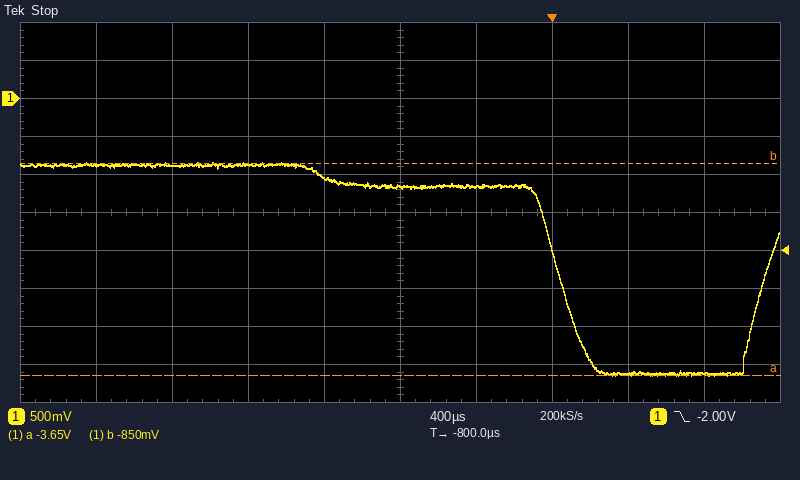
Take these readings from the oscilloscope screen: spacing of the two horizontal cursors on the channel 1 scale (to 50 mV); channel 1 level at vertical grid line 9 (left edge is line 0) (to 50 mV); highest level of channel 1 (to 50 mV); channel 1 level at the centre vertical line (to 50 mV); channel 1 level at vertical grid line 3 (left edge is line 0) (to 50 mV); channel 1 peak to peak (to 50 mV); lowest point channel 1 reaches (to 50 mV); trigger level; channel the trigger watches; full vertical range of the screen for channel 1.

2.80 V
-3.60 V
-850 mV
-1.15 V
-850 mV
2.80 V
-3.65 V
-2.00 V
channel 1
5 V
